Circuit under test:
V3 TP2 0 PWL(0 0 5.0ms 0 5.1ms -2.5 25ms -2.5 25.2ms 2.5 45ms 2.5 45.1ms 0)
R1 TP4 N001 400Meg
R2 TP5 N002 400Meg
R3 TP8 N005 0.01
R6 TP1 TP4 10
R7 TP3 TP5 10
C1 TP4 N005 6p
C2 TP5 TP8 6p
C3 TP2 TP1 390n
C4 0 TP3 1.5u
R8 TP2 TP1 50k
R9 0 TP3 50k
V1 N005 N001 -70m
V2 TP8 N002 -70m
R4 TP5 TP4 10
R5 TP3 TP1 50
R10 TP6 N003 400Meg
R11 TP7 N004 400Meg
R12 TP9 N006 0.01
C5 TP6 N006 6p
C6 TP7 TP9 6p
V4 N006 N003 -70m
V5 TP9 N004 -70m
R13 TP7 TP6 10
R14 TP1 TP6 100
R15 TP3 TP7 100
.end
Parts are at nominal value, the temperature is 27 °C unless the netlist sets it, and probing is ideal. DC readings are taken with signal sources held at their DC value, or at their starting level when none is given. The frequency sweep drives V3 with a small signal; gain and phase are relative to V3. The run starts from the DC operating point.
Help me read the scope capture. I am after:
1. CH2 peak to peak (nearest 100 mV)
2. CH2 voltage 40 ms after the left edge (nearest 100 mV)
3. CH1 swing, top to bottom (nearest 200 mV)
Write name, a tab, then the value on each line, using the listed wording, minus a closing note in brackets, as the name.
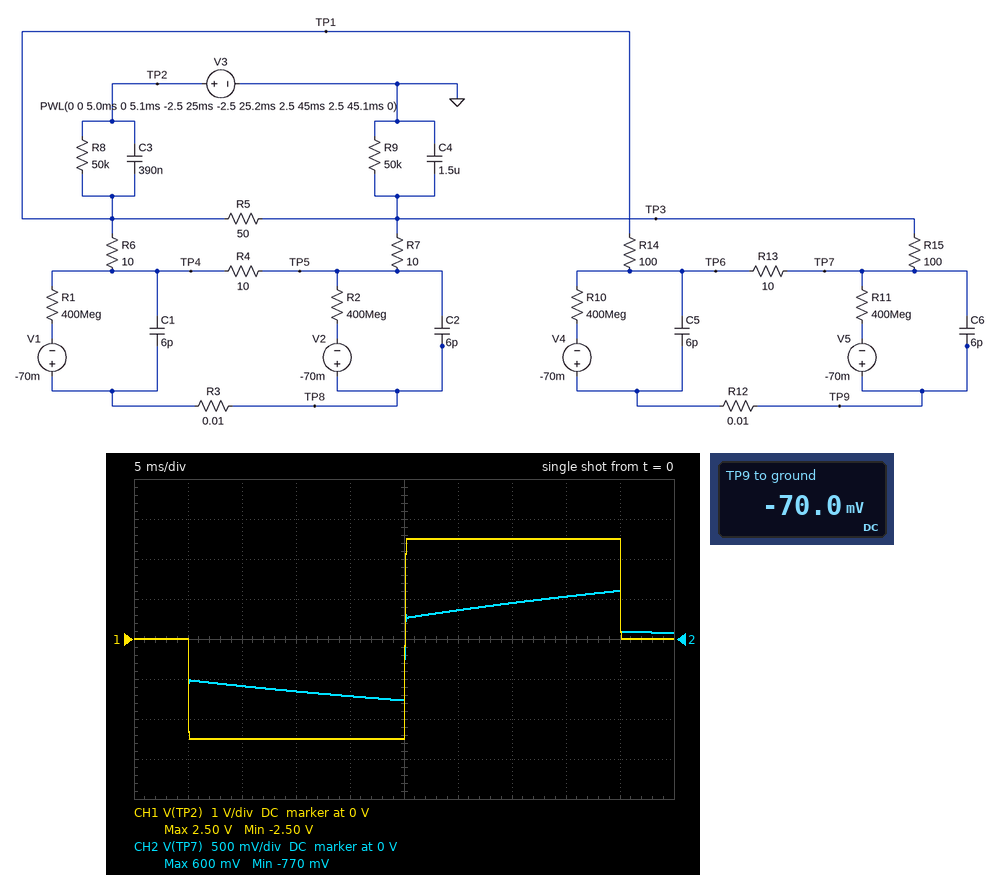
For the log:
CH2 peak to peak	1.4 V
CH2 voltage 40 ms after the left edge	500 mV
CH1 swing, top to bottom	5.0 V
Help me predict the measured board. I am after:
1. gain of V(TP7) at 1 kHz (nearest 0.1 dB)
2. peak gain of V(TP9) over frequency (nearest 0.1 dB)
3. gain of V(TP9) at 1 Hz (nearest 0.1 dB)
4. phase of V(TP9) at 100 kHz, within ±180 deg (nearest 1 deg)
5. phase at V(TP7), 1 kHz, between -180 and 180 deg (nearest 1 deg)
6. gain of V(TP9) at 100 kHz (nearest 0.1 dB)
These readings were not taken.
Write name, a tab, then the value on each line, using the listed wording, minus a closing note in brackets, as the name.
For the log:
gain of V(TP7) at 1 kHz	-13.7 dB
peak gain of V(TP9) over frequency	-6.0 dB
gain of V(TP9) at 1 Hz	-6.3 dB
phase of V(TP9) at 100 kHz, within ±180 deg	10 deg
phase at V(TP7), 1 kHz, between -180 and 180 deg	2 deg
gain of V(TP9) at 100 kHz	-6.3 dB
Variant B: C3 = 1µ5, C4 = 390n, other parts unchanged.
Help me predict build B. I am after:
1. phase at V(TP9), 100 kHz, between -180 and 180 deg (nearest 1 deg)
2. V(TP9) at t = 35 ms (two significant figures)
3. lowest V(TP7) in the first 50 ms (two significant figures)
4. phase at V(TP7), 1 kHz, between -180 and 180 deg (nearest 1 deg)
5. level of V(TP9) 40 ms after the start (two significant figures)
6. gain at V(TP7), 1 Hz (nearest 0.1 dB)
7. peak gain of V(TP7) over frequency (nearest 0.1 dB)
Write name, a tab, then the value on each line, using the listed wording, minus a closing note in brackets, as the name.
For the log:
phase at V(TP9), 100 kHz, between -180 and 180 deg	-9 deg
V(TP9) at t = 35 ms	2.0 V
lowest V(TP7) in the first 50 ms	-2.0 V
phase at V(TP7), 1 kHz, between -180 and 180 deg	-1 deg
level of V(TP9) 40 ms after the start	1.9 V
gain at V(TP7), 1 Hz	-5.5 dB
peak gain of V(TP7) over frequency	-2.0 dB
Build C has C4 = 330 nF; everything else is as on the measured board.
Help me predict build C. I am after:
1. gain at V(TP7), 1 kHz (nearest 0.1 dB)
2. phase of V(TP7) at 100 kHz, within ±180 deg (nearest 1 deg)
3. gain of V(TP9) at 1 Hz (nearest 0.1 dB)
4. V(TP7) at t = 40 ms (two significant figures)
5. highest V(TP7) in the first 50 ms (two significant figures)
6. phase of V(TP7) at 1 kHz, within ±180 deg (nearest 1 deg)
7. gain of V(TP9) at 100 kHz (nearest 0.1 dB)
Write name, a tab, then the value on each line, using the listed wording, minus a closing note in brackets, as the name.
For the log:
gain at V(TP7), 1 kHz	-5.3 dB
phase of V(TP7) at 100 kHz, within ±180 deg	-3 deg
gain of V(TP9) at 1 Hz	-6.0 dB
V(TP7) at t = 40 ms	1.3 V
highest V(TP7) in the first 50 ms	1.4 V
phase of V(TP7) at 1 kHz, within ±180 deg	0 deg
gain of V(TP9) at 100 kHz	-5.9 dB
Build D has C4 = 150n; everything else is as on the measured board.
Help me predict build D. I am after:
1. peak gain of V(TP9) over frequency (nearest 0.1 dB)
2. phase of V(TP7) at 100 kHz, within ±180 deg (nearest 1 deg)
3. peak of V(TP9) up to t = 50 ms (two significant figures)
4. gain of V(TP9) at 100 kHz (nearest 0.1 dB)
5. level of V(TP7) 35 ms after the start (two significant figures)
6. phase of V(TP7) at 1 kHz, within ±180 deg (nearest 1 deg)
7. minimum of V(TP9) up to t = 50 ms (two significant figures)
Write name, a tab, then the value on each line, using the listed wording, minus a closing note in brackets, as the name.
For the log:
peak gain of V(TP9) over frequency	-2.8 dB
phase of V(TP7) at 100 kHz, within ±180 deg	-12 deg
peak of V(TP9) up to t = 50 ms	2.2 V
gain of V(TP9) at 100 kHz	-4.4 dB
level of V(TP7) 35 ms after the start	1.7 V
phase of V(TP7) at 1 kHz, within ±180 deg	0 deg
minimum of V(TP9) up to t = 50 ms	-1.9 V
